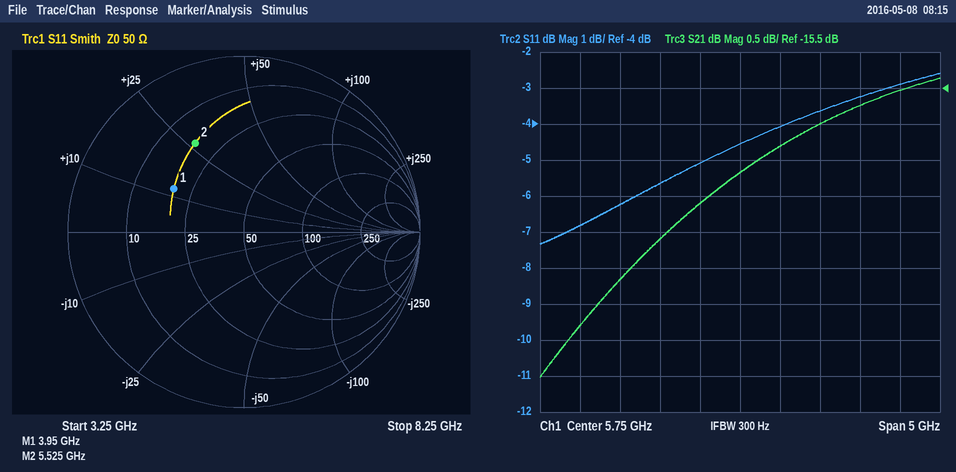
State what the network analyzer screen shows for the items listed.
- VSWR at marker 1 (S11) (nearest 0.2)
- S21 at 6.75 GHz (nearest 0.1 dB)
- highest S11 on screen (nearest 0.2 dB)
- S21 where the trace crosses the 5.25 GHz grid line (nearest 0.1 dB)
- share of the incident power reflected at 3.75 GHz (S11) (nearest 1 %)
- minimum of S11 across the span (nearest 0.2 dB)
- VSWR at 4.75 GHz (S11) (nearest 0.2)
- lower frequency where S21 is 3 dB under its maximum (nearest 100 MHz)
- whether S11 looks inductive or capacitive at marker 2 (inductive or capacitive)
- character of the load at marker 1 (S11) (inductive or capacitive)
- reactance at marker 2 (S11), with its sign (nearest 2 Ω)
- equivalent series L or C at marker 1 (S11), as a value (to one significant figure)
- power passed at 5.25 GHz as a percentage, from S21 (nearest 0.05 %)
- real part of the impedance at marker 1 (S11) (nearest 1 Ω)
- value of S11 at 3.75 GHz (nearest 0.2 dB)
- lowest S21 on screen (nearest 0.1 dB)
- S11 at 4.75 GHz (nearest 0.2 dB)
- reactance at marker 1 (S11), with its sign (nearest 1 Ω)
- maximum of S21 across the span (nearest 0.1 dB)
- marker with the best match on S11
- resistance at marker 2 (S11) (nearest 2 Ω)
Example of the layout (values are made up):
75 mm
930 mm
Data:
2.8
-16.0 dB
-2.6 dB
-17.1 dB
21 %
-7.4 dB
3.2
4.1 GHz
inductive
inductive
+26 Ω
500 pH
1.95 %
19 Ω
-6.8 dB
-19.5 dB
-5.6 dB
+12 Ω
-15.4 dB
marker 1
18 Ω
